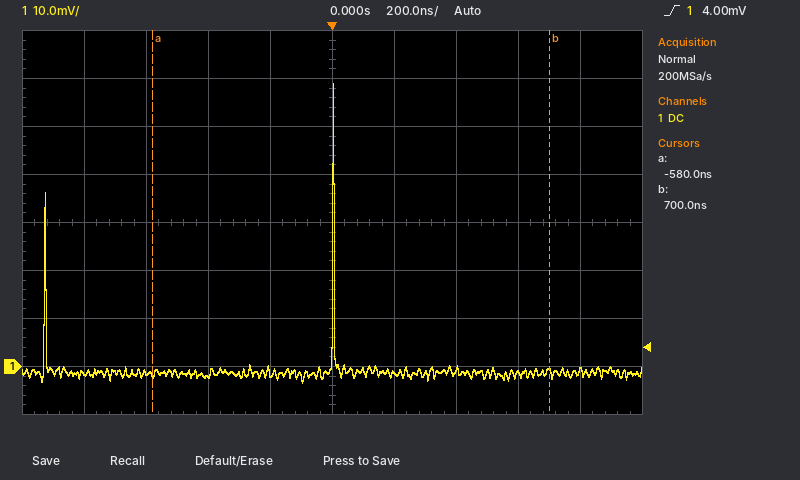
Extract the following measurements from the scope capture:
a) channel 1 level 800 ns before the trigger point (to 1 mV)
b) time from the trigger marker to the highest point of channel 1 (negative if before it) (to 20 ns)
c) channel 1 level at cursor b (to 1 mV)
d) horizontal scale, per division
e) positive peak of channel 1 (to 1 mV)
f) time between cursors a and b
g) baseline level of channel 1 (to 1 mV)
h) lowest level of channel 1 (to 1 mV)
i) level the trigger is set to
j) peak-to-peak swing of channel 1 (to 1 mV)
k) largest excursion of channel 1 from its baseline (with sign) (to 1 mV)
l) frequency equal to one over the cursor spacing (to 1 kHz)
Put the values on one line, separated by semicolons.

-1 mV; 0 ns; -1 mV; 200 ns; 59 mV; 1.28 µs; -1 mV; -3 mV; 4.00 mV; 62 mV; +60 mV; 781 kHz
